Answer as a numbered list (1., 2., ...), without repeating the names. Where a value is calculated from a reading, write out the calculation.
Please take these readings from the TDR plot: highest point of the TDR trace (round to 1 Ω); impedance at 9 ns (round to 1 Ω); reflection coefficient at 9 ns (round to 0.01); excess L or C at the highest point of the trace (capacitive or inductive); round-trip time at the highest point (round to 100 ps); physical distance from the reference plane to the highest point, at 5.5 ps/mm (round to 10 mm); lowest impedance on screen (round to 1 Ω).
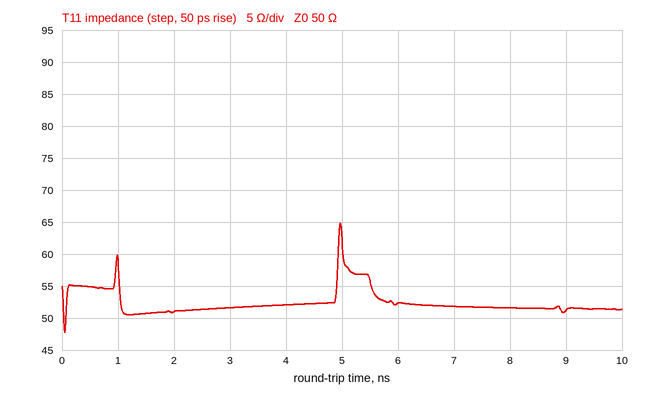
1. 65 Ω
2. 51 Ω
3. (51 − 50)/(51 + 50) ≈ +0.01
4. inductive
5. 5.0 ns
6. 5.0 ns / 2 / 5.5 ps/mm ≈ 455 mm, so 450 mm to the nearest 10 mm
7. 48 Ω
